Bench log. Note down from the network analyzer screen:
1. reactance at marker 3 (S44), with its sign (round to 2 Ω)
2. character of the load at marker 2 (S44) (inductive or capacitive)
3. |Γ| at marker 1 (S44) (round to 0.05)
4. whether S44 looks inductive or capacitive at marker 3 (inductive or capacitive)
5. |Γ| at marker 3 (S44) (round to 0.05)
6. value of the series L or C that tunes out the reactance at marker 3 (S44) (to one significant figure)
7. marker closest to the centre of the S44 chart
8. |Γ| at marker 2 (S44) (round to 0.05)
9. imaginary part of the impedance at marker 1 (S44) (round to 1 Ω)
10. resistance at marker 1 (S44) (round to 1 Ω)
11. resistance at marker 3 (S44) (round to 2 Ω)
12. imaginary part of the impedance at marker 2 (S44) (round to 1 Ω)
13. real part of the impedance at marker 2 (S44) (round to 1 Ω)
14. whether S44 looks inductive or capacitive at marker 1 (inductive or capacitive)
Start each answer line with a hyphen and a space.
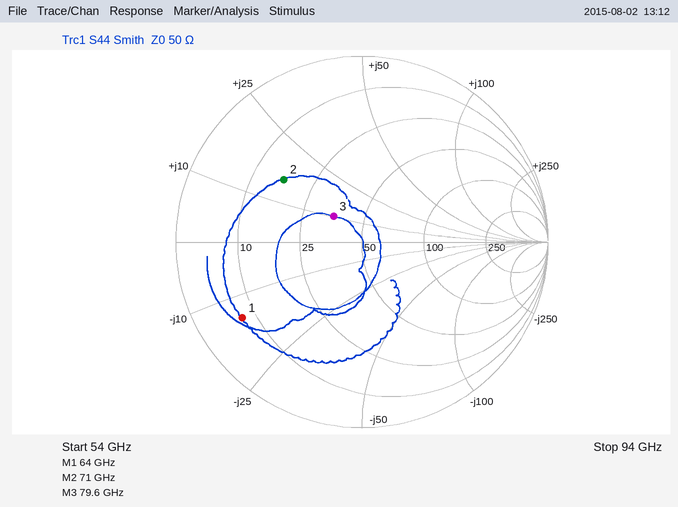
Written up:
- +10 Ω
- inductive
- 0.75
- inductive
- 0.20
- 200 fF
- marker 3
- 0.55
- -14 Ω
- 7 Ω
- 36 Ω
- +16 Ω
- 17 Ω
- capacitive
